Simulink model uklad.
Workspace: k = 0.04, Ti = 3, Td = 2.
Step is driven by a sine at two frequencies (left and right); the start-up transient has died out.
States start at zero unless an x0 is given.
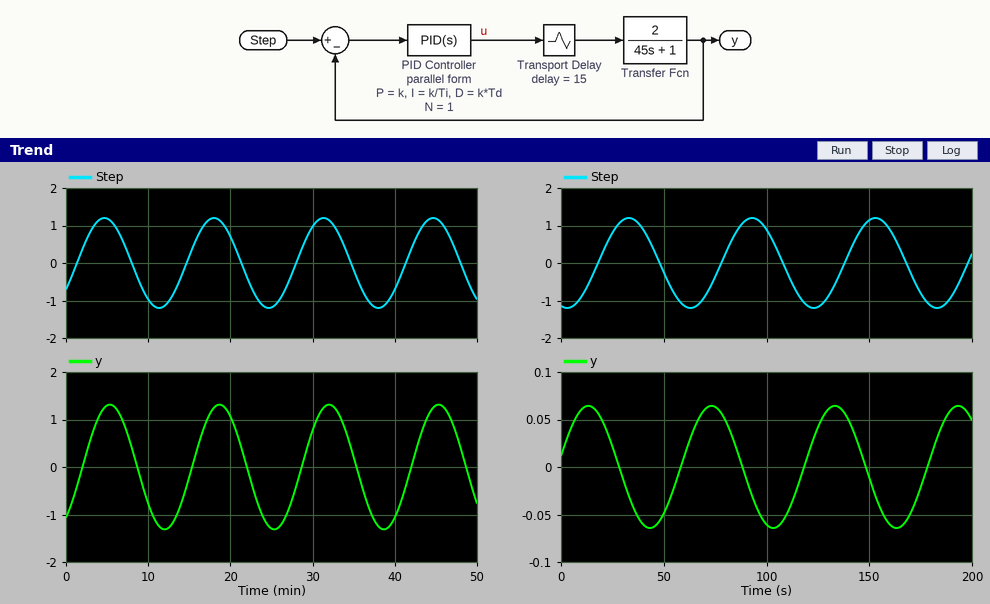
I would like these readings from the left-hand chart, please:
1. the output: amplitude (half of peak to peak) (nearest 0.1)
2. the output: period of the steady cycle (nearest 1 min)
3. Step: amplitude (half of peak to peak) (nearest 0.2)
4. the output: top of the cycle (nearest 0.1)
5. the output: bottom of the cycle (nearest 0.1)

1.3
13 min
1.2
1.3
-1.3
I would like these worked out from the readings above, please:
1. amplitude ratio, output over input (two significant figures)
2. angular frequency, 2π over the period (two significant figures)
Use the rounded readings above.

1.1
0.48 rad/min
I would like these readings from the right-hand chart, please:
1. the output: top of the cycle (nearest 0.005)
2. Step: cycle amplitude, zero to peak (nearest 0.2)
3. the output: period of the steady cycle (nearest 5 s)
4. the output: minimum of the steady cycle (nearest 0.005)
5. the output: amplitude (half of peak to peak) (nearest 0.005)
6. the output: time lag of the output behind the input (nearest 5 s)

0.065
1.2
60 s
-0.065
0.065
40 s
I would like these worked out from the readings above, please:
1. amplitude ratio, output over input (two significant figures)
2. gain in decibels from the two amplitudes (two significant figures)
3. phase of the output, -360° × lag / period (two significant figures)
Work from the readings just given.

0.054
-25 dB
-240°
